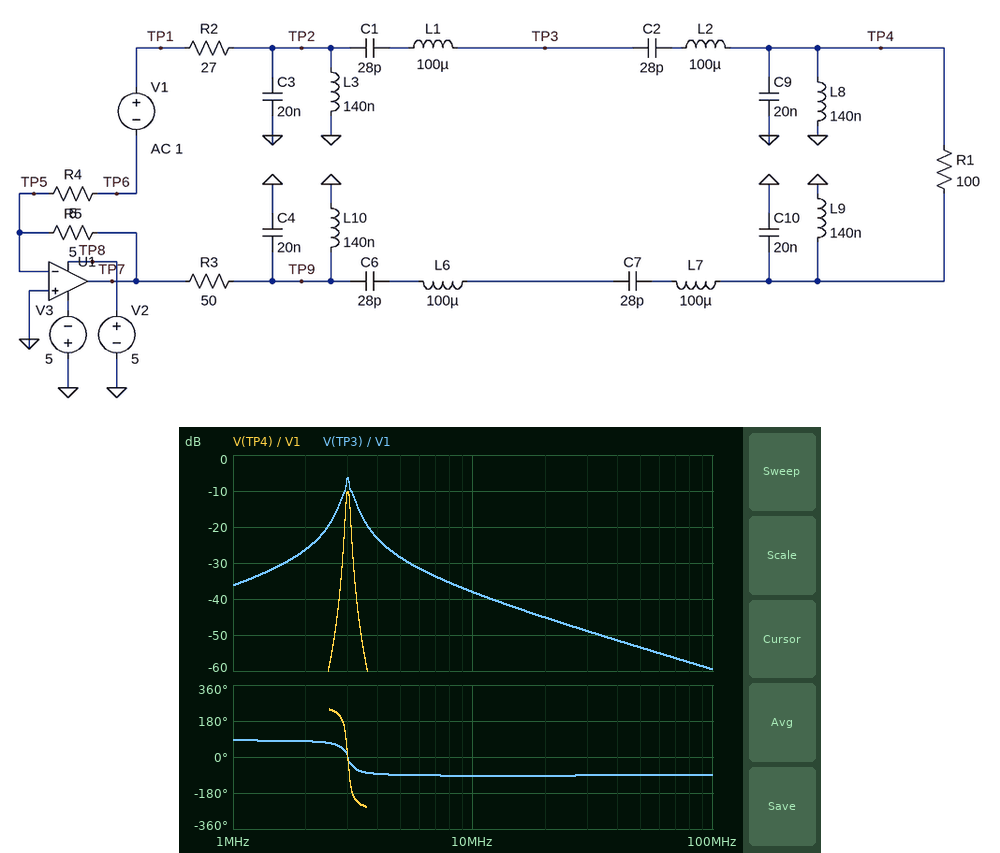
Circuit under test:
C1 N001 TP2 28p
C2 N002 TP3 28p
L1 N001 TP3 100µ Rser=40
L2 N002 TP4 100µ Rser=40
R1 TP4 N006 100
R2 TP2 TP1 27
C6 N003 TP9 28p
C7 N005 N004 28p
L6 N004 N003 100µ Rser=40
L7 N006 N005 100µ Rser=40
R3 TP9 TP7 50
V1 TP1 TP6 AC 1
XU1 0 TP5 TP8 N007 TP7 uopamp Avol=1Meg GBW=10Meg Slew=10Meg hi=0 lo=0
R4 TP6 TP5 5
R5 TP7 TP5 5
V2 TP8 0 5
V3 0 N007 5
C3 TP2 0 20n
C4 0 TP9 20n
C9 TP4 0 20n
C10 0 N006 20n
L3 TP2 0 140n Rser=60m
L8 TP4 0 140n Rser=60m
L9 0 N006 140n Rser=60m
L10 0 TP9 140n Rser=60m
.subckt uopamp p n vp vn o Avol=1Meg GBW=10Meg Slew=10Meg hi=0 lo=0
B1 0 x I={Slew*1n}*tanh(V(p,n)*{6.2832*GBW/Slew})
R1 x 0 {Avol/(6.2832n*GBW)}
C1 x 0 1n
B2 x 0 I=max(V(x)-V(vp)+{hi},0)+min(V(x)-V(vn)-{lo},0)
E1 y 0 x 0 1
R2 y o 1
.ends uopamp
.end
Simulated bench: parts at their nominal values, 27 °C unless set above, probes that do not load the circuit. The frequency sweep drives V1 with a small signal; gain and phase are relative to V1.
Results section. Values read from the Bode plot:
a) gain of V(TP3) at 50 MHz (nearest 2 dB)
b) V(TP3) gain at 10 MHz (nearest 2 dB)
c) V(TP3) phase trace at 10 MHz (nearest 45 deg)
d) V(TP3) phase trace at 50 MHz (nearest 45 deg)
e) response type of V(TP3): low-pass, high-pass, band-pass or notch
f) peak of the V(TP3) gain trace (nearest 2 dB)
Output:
-54 dB
-38 dB
-90 deg
-90 deg
band-pass
-6 dB
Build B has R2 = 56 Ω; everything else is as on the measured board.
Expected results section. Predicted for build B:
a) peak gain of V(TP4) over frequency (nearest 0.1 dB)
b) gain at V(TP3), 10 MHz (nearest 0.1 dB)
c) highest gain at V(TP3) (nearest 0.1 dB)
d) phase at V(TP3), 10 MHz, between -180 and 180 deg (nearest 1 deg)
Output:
-12.5 dB
-43.3 dB
-8.5 dB
-92 deg
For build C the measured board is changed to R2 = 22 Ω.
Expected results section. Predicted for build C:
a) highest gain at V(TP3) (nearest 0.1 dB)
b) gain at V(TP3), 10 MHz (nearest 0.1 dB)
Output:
-5.8 dB
-36.8 dB
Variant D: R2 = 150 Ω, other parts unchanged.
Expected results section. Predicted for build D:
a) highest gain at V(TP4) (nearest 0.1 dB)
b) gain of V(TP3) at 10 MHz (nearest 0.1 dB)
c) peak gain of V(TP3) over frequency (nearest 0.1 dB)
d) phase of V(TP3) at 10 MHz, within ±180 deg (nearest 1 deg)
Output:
-17.3 dB
-51.2 dB
-13.3 dB
-91 deg
